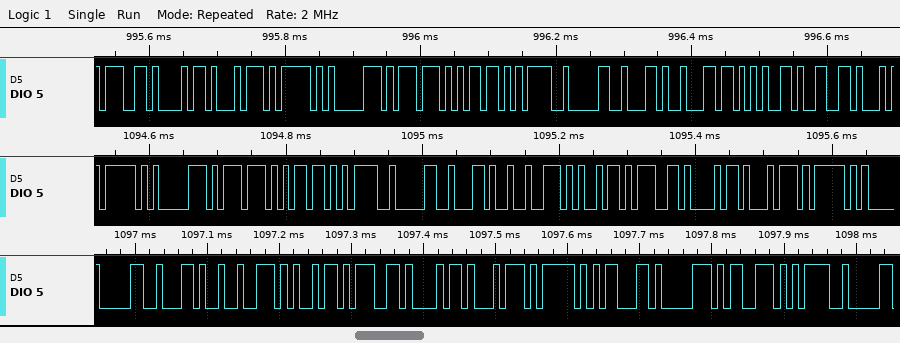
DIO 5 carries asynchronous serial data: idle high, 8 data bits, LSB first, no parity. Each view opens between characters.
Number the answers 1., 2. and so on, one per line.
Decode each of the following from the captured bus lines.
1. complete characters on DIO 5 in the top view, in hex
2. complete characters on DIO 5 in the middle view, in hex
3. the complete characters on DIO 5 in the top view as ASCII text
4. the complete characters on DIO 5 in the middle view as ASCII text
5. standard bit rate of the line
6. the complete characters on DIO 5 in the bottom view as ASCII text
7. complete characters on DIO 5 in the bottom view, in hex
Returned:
1. 67, 68, 74, 5F, 70, 77, 6D, 3D, 30, 2C, 6C, 65, 66
2. 5F, 70, 77, 6D, 3D, 30, 2C, 72, 69, 67, 68, 74, 5F
3. "ght_pwm=0,lef"
4. "_pwm=0,right_"
5. 115200 baud
6. "0,right_cps="
7. 30, 2C, 72, 69, 67, 68, 74, 5F, 63, 70, 73, 3D
